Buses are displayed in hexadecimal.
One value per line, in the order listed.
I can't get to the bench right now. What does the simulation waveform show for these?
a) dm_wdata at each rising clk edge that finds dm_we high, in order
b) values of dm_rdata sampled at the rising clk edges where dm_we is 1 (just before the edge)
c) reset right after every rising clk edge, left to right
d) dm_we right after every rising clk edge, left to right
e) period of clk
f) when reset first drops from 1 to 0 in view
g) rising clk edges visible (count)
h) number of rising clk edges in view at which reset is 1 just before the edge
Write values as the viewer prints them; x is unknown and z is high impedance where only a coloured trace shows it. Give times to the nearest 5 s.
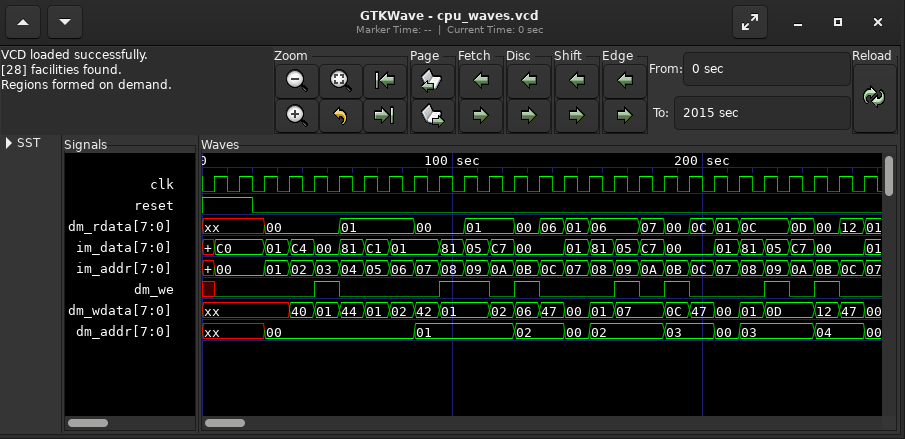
01, 01, 01, 06, 07, 0C, 0D, 12
00, 00, 01, 00, 06, 00, 0C, 00
1 1 0 0 0 0 0 0 0 0 0 0 0 0 0 0 0 0 0 0 0 0 0 0 0 0 0
0 0 0 0 1 0 0 0 0 1 1 0 1 0 0 0 1 0 1 0 0 0 1 0 1 0 0
10 s
20 s
27
2
